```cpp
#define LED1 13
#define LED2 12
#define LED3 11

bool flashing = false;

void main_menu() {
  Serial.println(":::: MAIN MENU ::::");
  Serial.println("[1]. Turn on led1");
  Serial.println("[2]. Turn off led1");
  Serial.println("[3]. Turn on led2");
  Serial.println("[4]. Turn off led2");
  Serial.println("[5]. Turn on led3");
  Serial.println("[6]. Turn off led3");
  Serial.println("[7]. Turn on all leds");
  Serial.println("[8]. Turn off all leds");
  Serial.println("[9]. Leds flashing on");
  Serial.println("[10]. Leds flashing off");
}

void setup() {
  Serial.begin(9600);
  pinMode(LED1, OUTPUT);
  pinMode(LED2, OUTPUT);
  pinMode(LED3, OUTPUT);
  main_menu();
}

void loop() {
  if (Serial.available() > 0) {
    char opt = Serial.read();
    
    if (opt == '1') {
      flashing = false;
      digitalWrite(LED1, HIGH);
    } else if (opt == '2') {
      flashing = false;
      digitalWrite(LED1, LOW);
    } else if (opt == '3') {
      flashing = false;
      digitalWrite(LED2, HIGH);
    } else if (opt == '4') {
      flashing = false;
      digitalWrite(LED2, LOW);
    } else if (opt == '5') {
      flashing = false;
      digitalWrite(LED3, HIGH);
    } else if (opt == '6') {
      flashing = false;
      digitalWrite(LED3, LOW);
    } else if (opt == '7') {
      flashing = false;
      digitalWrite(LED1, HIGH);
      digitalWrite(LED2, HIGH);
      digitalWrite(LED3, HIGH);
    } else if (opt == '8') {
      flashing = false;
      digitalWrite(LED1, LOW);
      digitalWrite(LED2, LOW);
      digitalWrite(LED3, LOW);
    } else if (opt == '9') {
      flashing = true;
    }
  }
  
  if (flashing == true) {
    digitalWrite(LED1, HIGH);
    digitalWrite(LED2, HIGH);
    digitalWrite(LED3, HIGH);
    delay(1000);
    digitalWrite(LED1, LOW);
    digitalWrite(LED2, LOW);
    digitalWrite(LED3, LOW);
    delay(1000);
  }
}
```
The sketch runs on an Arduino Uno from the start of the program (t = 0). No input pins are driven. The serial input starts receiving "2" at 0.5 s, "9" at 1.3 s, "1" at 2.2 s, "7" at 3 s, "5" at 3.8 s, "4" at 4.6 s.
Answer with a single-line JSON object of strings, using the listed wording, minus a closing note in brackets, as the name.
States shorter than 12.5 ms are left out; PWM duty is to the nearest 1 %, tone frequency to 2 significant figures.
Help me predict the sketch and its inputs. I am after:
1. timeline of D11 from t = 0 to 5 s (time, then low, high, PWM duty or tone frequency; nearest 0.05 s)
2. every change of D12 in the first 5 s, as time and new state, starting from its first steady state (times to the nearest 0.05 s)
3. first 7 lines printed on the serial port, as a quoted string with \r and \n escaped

{"timeline of D11 from t = 0 to 5 s": "0 s low; 1.3 s high; 2.3 s low; 3.3 s high", "every change of D12 in the first 5 s, as time and new state, starting from its first steady state": "0 s low; 1.3 s high; 2.3 s low; 3.3 s high; 4.6 s low", "first 7 lines printed on the serial port, as a quoted string with \\r and \\n escaped": "\":::: MAIN MENU ::::\\r\\n[1]. Turn on led1\\r\\n[2]. Turn off led1\\r\\n[3]. Turn on led2\\r\\n[4]. Turn off led2\\r\\n[5]. Turn on led3\\r\\n[6]. Turn off led3\\r\\n\""}
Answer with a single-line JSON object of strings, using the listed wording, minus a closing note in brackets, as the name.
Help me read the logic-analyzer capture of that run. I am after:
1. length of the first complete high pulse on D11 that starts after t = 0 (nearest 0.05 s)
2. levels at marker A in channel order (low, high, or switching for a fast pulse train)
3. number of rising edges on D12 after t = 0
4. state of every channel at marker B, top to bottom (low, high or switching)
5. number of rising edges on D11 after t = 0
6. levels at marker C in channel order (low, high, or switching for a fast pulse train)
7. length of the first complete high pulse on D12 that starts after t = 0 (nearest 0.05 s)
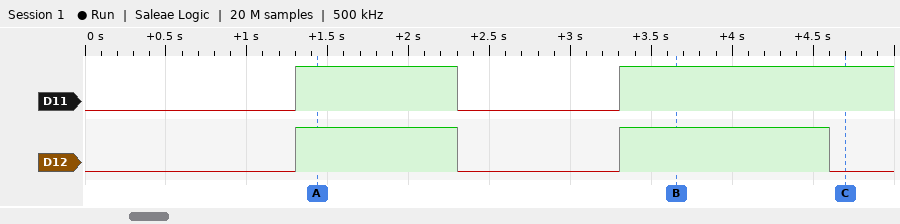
{"length of the first complete high pulse on D11 that starts after t = 0": "1.00 s", "levels at marker A in channel order": "D11 high, D12 high", "number of rising edges on D12 after t = 0": "2", "state of every channel at marker B, top to bottom": "D11 high, D12 high", "number of rising edges on D11 after t = 0": "2", "levels at marker C in channel order": "D11 high, D12 low", "length of the first complete high pulse on D12 that starts after t = 0": "1.00 s"}
